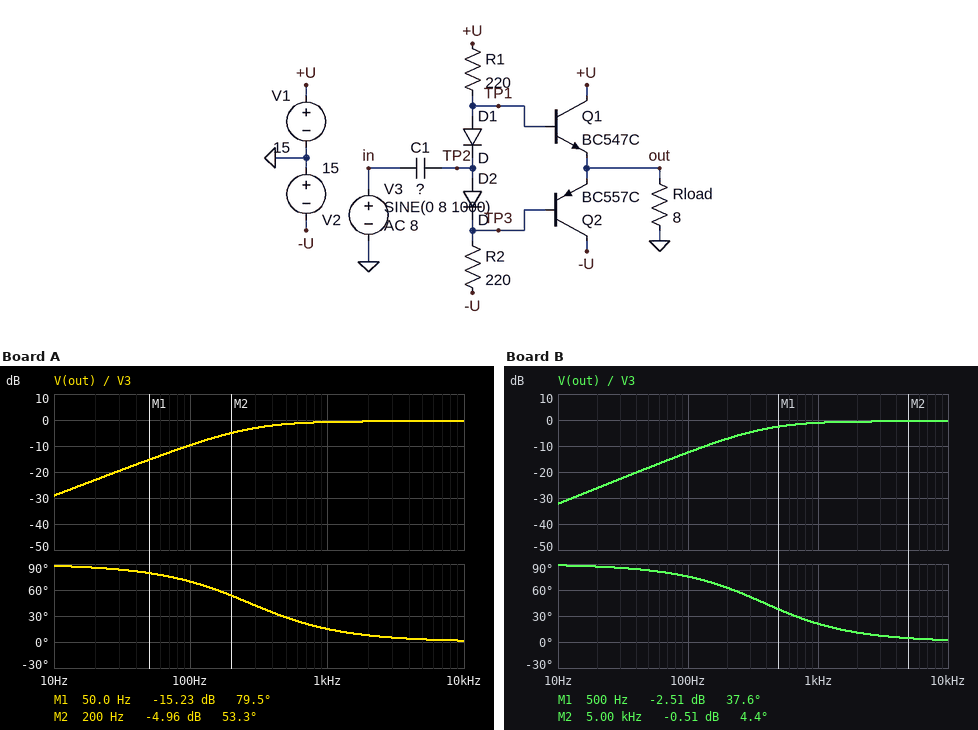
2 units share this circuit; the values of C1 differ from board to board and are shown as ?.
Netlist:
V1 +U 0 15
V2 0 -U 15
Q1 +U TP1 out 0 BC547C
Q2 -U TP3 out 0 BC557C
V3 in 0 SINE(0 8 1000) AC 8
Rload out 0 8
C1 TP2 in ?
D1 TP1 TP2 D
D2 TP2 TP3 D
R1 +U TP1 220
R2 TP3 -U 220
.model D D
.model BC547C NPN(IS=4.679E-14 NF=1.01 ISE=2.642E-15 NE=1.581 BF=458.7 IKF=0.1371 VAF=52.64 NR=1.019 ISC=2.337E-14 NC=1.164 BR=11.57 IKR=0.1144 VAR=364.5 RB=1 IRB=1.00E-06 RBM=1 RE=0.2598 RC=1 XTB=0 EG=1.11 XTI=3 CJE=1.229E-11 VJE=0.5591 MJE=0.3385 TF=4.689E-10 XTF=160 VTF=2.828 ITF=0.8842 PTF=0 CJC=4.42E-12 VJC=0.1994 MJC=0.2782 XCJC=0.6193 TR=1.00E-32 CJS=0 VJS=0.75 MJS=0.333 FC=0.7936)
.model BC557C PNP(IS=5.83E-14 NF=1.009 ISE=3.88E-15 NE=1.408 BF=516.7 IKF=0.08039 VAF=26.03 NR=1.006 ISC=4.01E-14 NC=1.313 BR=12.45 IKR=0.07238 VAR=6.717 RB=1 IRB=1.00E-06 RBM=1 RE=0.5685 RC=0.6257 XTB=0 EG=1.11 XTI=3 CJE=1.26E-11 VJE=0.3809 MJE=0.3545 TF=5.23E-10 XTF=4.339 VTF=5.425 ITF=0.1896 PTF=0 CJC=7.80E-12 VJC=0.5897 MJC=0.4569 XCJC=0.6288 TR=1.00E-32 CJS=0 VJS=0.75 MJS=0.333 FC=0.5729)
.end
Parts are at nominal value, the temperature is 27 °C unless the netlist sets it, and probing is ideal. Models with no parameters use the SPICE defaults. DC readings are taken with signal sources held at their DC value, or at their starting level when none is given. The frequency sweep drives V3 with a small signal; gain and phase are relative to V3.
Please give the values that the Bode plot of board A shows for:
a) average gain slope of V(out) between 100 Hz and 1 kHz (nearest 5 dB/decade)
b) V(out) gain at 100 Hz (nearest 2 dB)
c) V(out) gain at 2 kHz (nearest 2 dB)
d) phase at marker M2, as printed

10 dB/decade
-10 dB
0 dB
53.3 deg
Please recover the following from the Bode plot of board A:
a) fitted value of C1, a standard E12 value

5.6 µF
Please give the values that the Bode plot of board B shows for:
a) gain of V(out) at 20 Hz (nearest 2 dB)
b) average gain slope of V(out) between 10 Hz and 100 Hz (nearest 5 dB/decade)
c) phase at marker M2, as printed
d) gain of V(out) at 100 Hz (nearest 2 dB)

-26 dB
20 dB/decade
4.4 deg
-12 dB
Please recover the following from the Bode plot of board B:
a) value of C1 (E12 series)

3.9 µF
